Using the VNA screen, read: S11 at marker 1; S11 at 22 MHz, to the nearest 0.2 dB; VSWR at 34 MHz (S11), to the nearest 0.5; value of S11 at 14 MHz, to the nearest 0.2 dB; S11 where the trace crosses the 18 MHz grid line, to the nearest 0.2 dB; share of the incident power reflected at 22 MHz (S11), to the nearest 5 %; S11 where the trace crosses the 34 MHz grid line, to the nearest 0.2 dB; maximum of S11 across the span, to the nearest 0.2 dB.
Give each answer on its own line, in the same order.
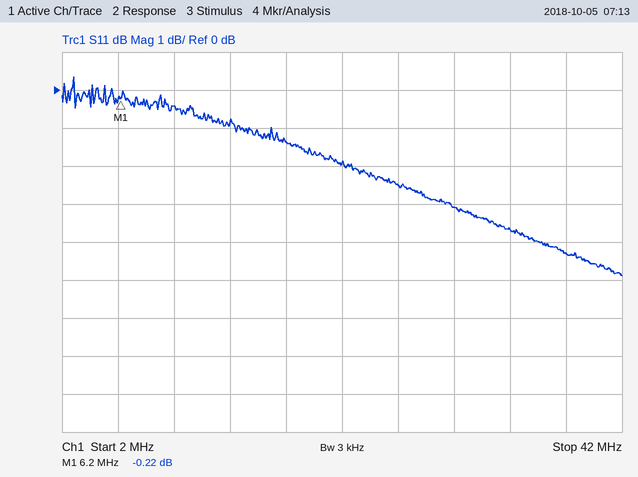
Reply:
-0.22 dB
-2.0 dB
5.0
-0.8 dB
-1.4 dB
65 %
-3.6 dB
0.4 dB
